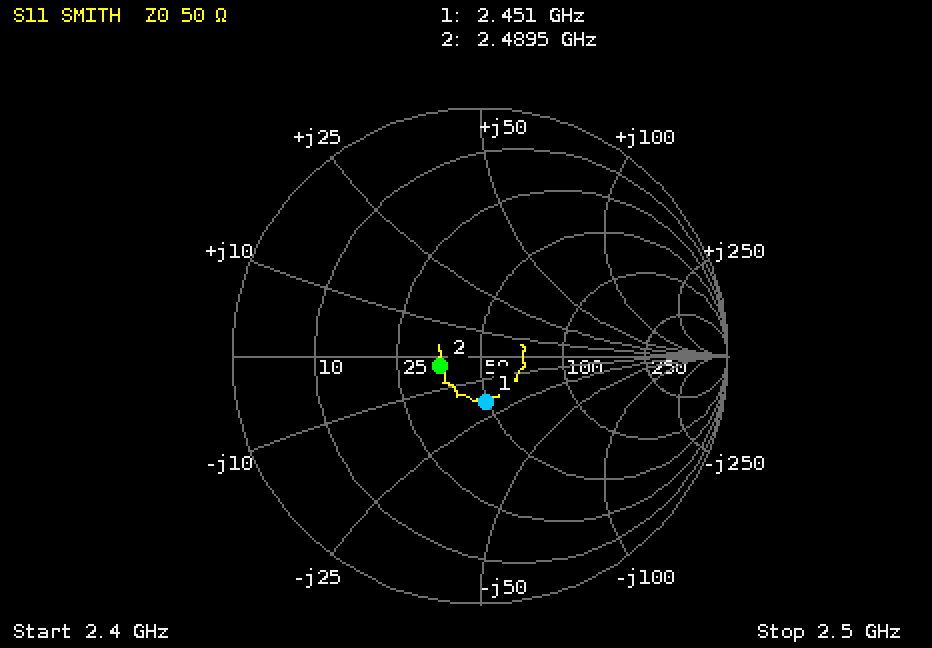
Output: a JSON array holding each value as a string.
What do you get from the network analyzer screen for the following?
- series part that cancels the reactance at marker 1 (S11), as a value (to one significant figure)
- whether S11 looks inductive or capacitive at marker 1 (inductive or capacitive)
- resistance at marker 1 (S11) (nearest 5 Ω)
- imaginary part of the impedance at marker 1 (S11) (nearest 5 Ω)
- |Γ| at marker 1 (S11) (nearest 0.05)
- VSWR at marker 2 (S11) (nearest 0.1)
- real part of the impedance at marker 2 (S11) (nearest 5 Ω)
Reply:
["1 nH", "capacitive", "50 Ω", "-20 Ω", "0.20", "1.4", "35 Ω"]
